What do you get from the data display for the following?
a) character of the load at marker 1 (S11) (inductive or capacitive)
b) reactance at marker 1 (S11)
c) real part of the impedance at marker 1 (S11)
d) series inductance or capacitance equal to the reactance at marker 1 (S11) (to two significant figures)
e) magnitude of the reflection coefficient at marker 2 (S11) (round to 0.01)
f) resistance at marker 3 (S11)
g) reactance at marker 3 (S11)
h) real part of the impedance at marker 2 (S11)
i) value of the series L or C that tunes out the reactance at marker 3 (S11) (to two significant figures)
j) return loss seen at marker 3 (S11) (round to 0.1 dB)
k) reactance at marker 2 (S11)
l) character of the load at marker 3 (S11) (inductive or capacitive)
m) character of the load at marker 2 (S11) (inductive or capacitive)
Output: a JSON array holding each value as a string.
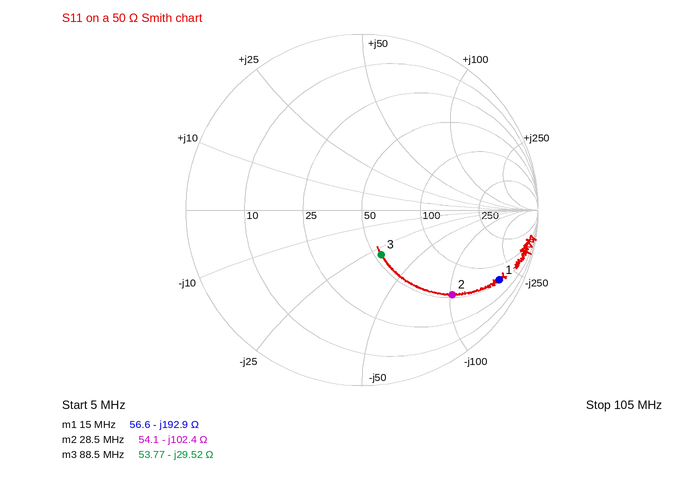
["capacitive", "-192.9 Ω", "56.6 Ω", "55 pF", "0.70", "53.77 Ω", "-29.52 Ω", "54.1 Ω", "53 nH", "11.2 dB", "-102.4 Ω", "capacitive", "capacitive"]
